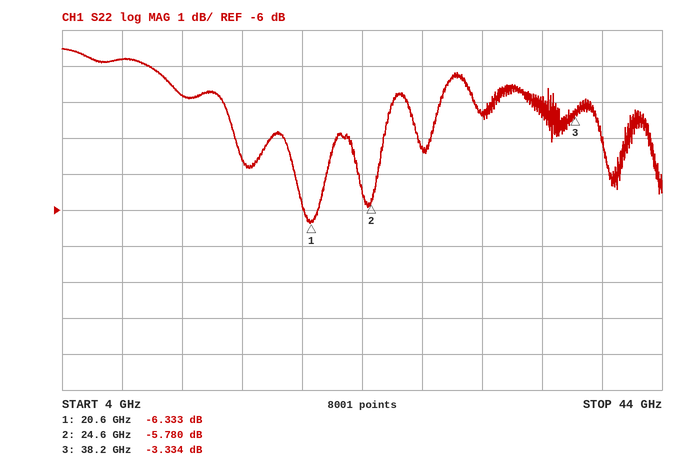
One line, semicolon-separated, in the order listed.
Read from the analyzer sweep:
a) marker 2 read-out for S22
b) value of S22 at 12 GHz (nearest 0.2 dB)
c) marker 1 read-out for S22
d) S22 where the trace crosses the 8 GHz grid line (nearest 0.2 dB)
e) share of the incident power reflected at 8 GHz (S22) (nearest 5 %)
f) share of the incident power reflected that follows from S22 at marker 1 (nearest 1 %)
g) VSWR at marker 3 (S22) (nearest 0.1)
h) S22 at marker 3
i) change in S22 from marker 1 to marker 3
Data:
-5.780 dB; -2.8 dB; -6.333 dB; -1.8 dB; 65 %; 23 %; 5.3; -3.334 dB; 2.999 dB
